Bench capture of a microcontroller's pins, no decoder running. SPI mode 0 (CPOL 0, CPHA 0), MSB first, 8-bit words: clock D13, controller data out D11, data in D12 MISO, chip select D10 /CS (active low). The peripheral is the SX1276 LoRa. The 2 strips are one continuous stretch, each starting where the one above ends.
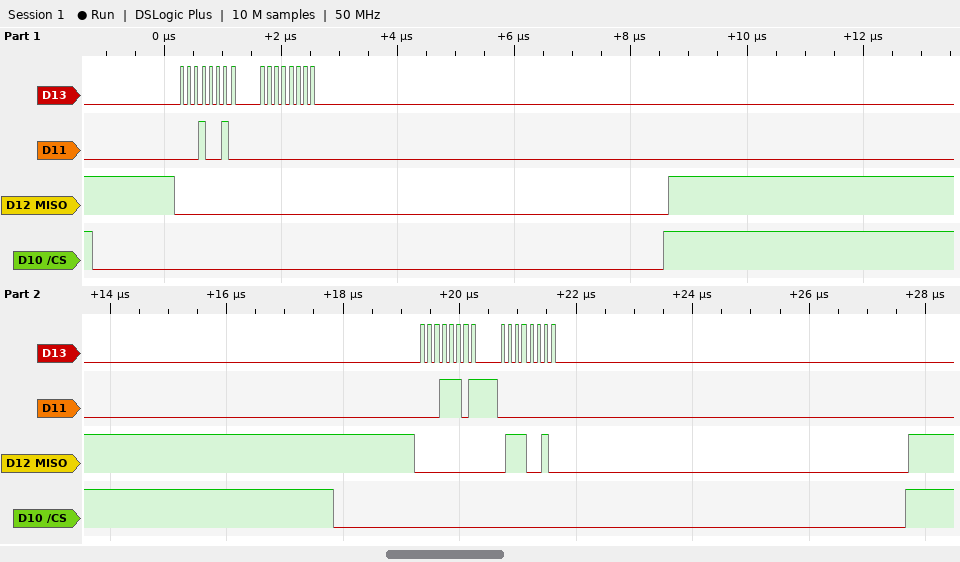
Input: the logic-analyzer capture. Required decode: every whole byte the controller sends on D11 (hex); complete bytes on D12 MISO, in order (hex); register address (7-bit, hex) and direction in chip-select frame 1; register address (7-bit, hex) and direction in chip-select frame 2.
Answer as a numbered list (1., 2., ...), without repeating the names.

1. 0x12 0x00 0x1D 0x00
2. 0x00 0x00 0x00 0x72
3. 0x12 read
4. 0x1D read
